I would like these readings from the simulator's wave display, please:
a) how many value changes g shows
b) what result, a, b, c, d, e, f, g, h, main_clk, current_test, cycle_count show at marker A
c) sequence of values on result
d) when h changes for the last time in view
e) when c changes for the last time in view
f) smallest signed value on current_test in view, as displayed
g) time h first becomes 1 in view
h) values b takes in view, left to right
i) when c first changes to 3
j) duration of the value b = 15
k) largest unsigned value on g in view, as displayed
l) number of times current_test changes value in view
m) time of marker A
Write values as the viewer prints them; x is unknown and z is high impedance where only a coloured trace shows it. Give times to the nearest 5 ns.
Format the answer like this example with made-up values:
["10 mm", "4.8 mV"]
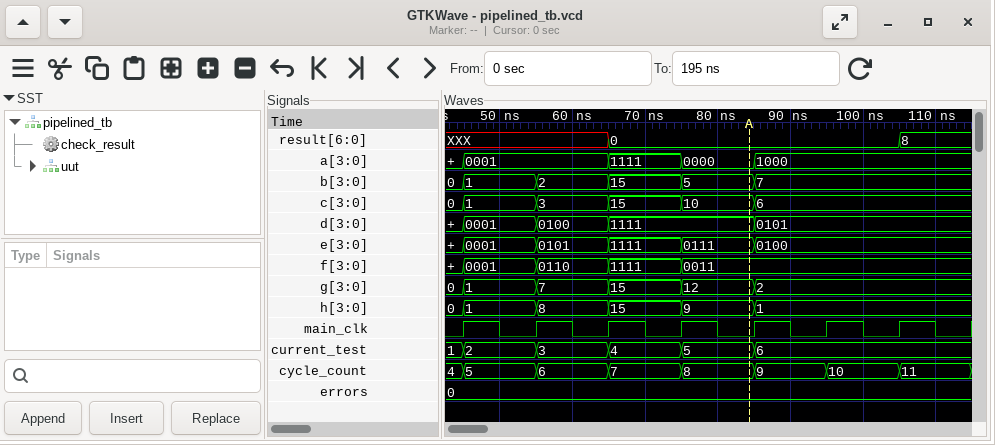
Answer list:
["5", "result=0, a=0000, b=5, c=10, d=1111, e=0111, f=0011, g=12, h=9, main_clk=0, current_test=5, cycle_count=8", "XXX, 0, 8", "85 ns", "85 ns", "1", "45 ns", "0, 1, 2, 15, 5, 7", "55 ns", "10 ns", "15", "5", "85 ns"]
